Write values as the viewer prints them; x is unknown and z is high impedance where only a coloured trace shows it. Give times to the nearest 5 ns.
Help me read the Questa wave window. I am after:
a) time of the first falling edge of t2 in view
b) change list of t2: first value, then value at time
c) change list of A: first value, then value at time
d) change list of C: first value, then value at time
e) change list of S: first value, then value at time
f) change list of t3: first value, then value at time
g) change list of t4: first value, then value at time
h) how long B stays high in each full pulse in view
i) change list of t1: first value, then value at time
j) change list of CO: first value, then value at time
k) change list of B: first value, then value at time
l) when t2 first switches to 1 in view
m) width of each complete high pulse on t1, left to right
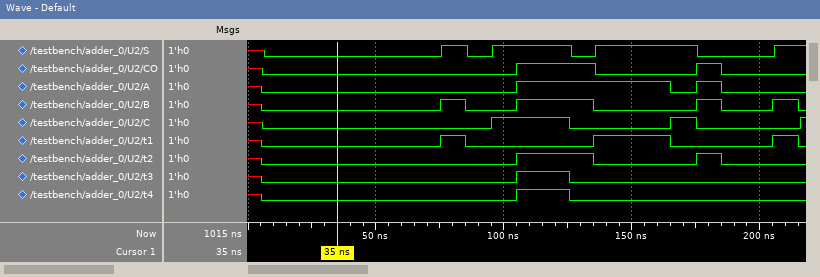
135 ns
x, 0 at 5 ns, 1 at 105 ns, 0 at 135 ns, 1 at 175 ns, 0 at 185 ns
x, 0 at 5 ns, 1 at 105 ns, 0 at 165 ns, 1 at 175 ns, 0 at 185 ns
x, 0 at 5 ns, 1 at 95 ns, 0 at 125 ns, 1 at 165 ns, 0 at 175 ns, 1 at 215 ns
x, 0 at 5 ns, 1 at 75 ns, 0 at 85 ns, 1 at 95 ns, 0 at 125 ns, 1 at 135 ns, 0 at 175 ns, 1 at 205 ns
x, 0 at 5 ns, 1 at 105 ns, 0 at 125 ns
x, 0 at 5 ns, 1 at 105 ns, 0 at 125 ns
10 ns, 30 ns, 10 ns, 10 ns
x, 0 at 5 ns, 1 at 75 ns, 0 at 85 ns, 1 at 135 ns, 0 at 165 ns, 1 at 205 ns, 0 at 215 ns
x, 0 at 5 ns, 1 at 105 ns, 0 at 135 ns, 1 at 175 ns, 0 at 185 ns
x, 0 at 5 ns, 1 at 75 ns, 0 at 85 ns, 1 at 105 ns, 0 at 135 ns, 1 at 175 ns, 0 at 185 ns, 1 at 205 ns, 0 at 215 ns
105 ns
10 ns, 30 ns, 10 ns
